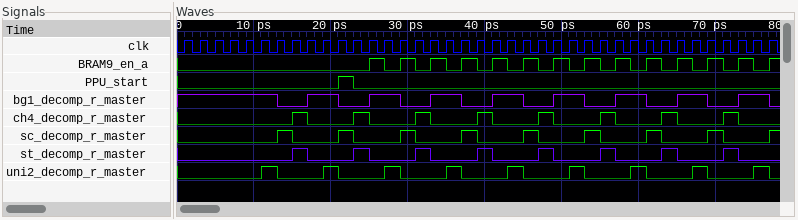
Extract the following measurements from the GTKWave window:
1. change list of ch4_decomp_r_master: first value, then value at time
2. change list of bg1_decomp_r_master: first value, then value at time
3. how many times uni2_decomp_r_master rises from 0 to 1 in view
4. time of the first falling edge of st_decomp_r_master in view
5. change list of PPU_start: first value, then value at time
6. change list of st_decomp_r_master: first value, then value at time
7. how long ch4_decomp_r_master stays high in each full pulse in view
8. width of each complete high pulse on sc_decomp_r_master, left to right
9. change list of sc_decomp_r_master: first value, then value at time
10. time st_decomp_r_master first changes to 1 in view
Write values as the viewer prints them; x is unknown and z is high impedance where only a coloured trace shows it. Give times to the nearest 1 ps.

0, 1 at 15 ps, 0 at 17 ps, 1 at 23 ps, 0 at 25 ps, 1 at 31 ps, 0 at 33 ps, 1 at 39 ps, 0 at 41 ps, 1 at 47 ps, 0 at 49 ps, 1 at 55 ps, 0 at 57 ps, 1 at 63 ps, 0 at 65 ps, 1 at 71 ps, 0 at 73 ps
1, 0 at 13 ps, 1 at 17 ps, 0 at 21 ps, 1 at 25 ps, 0 at 29 ps, 1 at 33 ps, 0 at 37 ps, 1 at 41 ps, 0 at 45 ps, 1 at 49 ps, 0 at 53 ps, 1 at 57 ps, 0 at 61 ps, 1 at 65 ps, 0 at 69 ps, 1 at 73 ps, 0 at 77 ps
9
17 ps
0, 1 at 21 ps, 0 at 23 ps
0, 1 at 15 ps, 0 at 17 ps, 1 at 23 ps, 0 at 25 ps, 1 at 31 ps, 0 at 33 ps, 1 at 39 ps, 0 at 41 ps, 1 at 47 ps, 0 at 49 ps, 1 at 55 ps, 0 at 57 ps, 1 at 63 ps, 0 at 65 ps, 1 at 71 ps, 0 at 73 ps
2 ps, 2 ps, 2 ps, 2 ps, 2 ps, 2 ps, 2 ps, 2 ps
2 ps, 2 ps, 2 ps, 2 ps, 2 ps, 2 ps, 2 ps, 2 ps
0, 1 at 13 ps, 0 at 15 ps, 1 at 21 ps, 0 at 23 ps, 1 at 29 ps, 0 at 31 ps, 1 at 37 ps, 0 at 39 ps, 1 at 45 ps, 0 at 47 ps, 1 at 53 ps, 0 at 55 ps, 1 at 61 ps, 0 at 63 ps, 1 at 69 ps, 0 at 71 ps, 1 at 77 ps
15 ps
